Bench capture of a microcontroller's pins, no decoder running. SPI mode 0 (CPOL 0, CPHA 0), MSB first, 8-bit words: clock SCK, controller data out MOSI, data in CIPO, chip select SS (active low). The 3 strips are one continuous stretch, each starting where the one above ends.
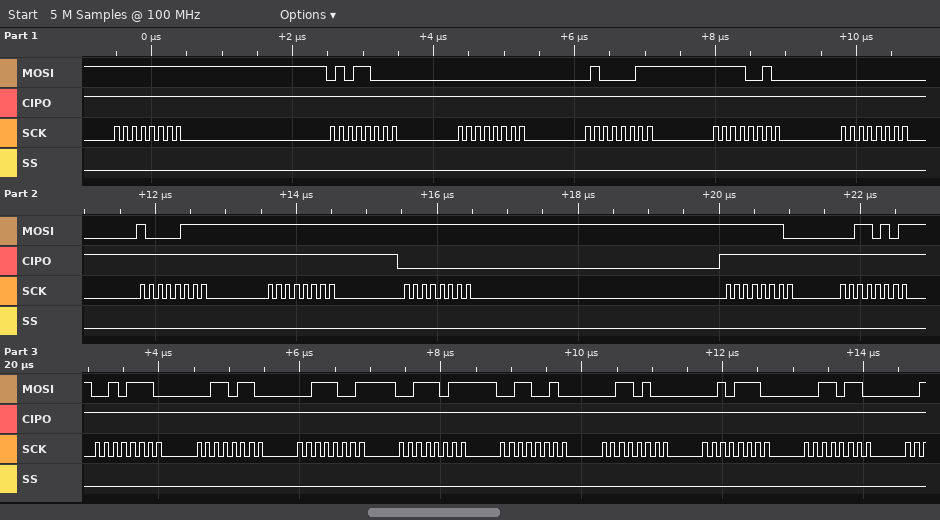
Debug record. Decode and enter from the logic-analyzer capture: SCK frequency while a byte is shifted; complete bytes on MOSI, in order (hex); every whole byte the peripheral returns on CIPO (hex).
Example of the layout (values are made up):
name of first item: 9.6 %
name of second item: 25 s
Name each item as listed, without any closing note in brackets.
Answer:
SCK frequency while a byte is shifted: 8 MHz
complete bytes on MOSI, in order: 0xFF 0x58 0x00 0x43 0xF2 0x00 0x87 0xFF 0xFF 0xFE 0x35 0x2E 0x36 0x39 0x3B 0x32 0x34 0x2E 0x36
every whole byte the peripheral returns on CIPO: 0xFF 0xFF 0xFF 0xFF 0xFF 0xFF 0xFF 0xFF 0x00 0xFF 0xFF 0xFF 0xFF 0xFF 0xFF 0xFF 0xFF 0xFF 0xFF
